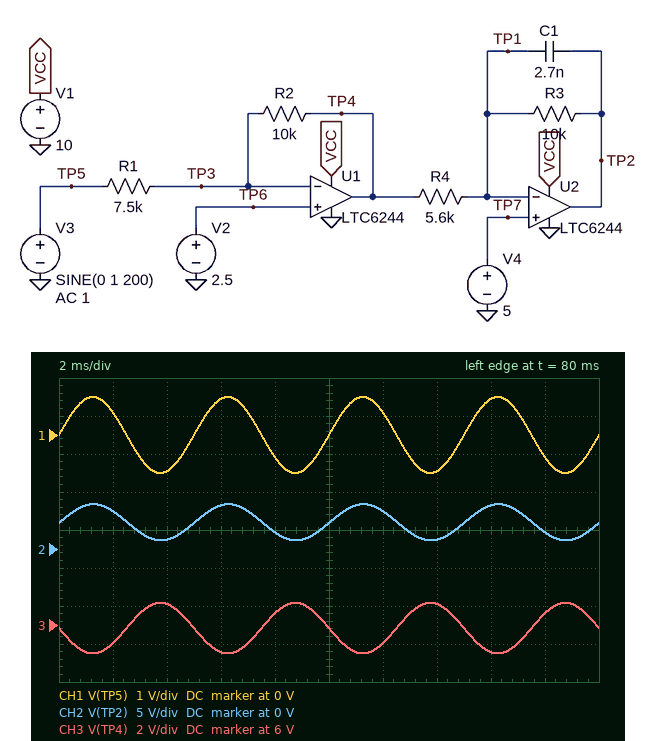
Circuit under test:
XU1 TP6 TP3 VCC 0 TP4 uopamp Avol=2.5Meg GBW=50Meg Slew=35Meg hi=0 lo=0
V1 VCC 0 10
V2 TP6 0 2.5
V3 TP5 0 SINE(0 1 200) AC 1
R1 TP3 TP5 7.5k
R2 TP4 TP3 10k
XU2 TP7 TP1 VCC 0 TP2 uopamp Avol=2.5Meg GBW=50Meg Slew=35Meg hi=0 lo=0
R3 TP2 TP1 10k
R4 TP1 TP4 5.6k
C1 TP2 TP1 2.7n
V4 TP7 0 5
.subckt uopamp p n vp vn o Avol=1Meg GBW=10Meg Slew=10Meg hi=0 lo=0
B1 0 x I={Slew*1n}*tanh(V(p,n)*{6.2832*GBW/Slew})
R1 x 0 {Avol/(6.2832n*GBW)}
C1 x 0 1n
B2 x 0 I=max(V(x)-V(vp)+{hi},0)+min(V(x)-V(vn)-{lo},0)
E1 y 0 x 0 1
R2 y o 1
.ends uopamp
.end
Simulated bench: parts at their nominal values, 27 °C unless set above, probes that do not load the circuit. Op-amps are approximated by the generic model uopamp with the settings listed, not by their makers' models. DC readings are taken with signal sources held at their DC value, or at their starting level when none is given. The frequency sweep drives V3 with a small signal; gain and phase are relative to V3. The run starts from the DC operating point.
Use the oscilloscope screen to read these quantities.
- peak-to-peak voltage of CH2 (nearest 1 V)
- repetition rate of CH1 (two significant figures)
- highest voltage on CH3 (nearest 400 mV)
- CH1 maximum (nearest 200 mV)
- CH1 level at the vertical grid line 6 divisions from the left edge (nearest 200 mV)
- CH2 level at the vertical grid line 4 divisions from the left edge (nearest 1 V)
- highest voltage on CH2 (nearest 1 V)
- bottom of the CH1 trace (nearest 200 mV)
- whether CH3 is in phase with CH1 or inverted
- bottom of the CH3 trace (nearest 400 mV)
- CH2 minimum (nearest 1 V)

5 V
200 Hz
7.2 V
1.0 V
600 mV
2 V
6 V
-1.0 V
inverted
4.4 V
1 V
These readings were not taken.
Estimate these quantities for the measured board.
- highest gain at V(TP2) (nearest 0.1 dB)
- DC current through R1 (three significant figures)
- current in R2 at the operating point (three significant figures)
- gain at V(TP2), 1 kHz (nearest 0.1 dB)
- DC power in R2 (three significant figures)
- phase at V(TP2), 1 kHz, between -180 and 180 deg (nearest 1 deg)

7.5 dB
333 µA
333 µA
7.4 dB
1.11 mW
-10 deg
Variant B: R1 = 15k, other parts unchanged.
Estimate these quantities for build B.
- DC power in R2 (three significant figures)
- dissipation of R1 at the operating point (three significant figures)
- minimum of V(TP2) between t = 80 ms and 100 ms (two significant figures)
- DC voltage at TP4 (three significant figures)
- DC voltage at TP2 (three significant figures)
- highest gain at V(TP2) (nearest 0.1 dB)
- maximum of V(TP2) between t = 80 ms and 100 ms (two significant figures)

278 µW
417 µW
5.3 V
4.17 V
6.49 V
1.5 dB
7.7 V
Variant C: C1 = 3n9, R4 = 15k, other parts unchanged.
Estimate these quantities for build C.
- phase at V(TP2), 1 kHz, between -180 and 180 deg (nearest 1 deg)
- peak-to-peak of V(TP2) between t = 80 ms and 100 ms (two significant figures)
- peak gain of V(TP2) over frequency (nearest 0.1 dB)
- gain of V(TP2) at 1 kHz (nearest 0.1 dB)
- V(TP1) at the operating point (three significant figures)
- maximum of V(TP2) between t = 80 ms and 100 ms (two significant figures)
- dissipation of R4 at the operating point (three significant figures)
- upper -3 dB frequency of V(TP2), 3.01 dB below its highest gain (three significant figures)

-14 deg
1.8 V
-1.0 dB
-1.3 dB
5.00 V
5.3 V
46.3 µW
4.08 kHz
